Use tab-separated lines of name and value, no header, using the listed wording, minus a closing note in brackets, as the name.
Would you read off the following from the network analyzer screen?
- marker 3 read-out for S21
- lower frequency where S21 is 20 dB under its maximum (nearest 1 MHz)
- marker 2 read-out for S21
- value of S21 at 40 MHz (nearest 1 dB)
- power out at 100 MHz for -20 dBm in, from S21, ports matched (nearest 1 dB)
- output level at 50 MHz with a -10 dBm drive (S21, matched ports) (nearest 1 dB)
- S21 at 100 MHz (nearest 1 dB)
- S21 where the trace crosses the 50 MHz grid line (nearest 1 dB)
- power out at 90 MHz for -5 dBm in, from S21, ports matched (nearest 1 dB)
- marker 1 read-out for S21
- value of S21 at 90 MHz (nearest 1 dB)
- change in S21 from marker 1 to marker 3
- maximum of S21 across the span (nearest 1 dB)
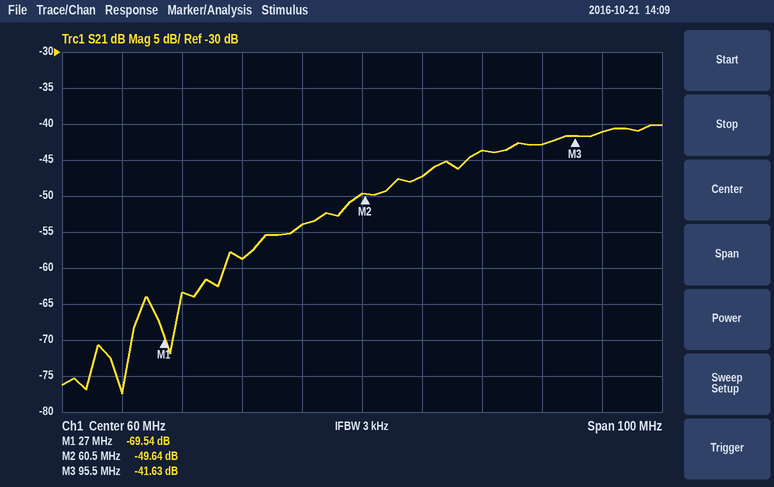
marker 3 read-out for S21	-41.63 dB
lower frequency where S21 is 20 dB under its maximum	37 MHz
marker 2 read-out for S21	-49.64 dB
value of S21 at 40 MHz	-59 dB
power out at 100 MHz for -20 dBm in, from S21, ports matched	-61 dBm
output level at 50 MHz with a -10 dBm drive (S21, matched ports)	-64 dBm
S21 at 100 MHz	-41 dB
S21 where the trace crosses the 50 MHz grid line	-54 dB
power out at 90 MHz for -5 dBm in, from S21, ports matched	-48 dBm
marker 1 read-out for S21	-69.54 dB
value of S21 at 90 MHz	-43 dB
change in S21 from marker 1 to marker 3	27.91 dB
maximum of S21 across the span	-40 dB
